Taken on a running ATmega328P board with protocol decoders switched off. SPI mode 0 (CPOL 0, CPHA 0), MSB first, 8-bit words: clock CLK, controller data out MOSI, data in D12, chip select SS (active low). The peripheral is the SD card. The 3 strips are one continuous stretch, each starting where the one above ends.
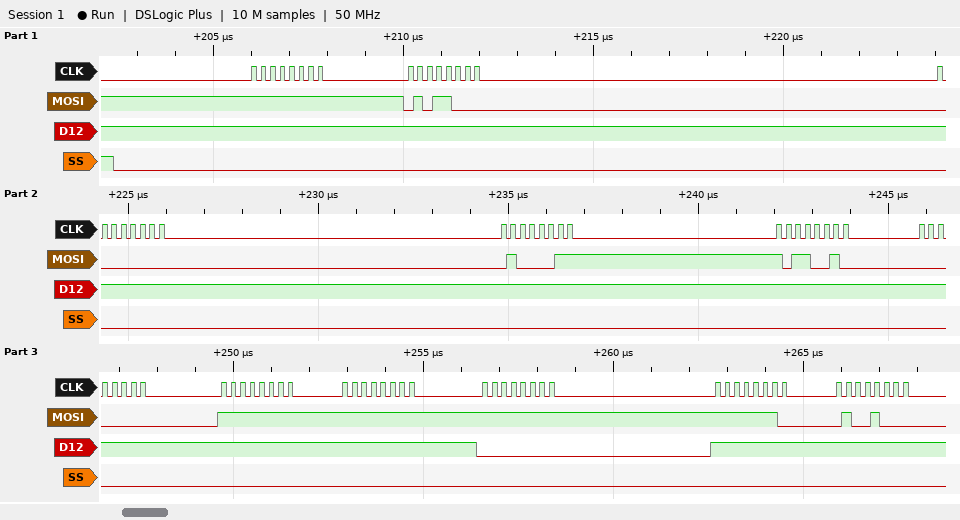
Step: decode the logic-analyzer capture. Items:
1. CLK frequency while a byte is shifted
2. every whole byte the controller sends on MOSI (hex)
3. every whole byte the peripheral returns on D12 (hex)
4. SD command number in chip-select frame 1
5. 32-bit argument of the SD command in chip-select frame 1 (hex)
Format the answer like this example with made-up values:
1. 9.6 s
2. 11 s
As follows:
1. 4 MHz
2. FF 58 00 43 B2 00 FF FF FF FE 48
3. FF FF FF FF FF FF FF FF 00 FF FF
4. CMD24
5. 0x0043B200
